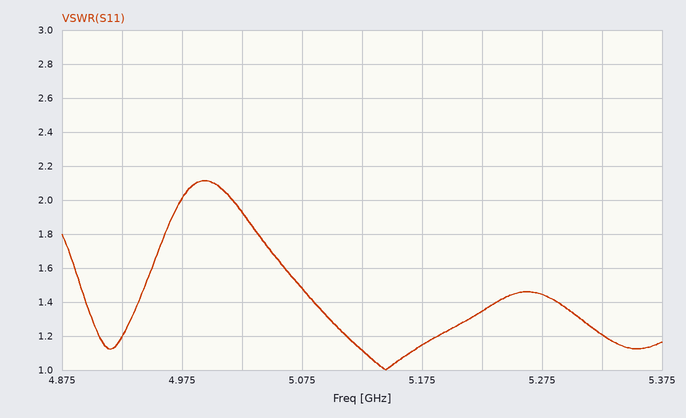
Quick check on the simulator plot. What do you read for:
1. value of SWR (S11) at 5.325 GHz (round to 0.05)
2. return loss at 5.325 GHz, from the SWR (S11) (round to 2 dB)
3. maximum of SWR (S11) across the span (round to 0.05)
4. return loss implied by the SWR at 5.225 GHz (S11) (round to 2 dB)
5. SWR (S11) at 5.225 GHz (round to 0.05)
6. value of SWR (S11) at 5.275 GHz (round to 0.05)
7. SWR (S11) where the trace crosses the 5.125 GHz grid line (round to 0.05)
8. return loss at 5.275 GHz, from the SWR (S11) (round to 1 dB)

1.20
20 dB
2.10
16 dB
1.35
1.45
1.10
15 dB
